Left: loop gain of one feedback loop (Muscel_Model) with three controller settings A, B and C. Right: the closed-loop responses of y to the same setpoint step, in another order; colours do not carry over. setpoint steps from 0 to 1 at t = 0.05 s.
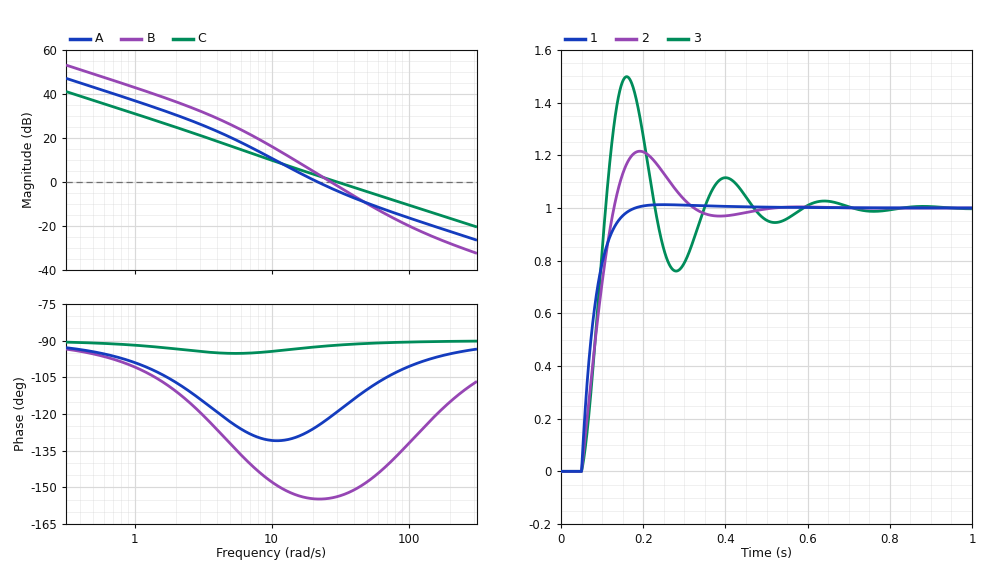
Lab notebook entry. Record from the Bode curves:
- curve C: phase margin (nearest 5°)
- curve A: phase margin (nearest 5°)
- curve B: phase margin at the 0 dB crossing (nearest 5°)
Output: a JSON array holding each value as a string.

["90°", "55°", "25°"]
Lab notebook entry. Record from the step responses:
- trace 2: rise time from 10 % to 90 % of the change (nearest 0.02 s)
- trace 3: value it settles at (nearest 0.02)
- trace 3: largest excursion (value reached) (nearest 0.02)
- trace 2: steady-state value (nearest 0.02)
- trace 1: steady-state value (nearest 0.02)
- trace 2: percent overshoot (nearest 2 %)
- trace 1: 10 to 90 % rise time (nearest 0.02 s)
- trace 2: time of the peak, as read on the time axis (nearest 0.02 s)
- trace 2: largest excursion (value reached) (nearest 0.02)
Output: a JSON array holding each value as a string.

["0.06 s", "1.00", "1.50", "1.00", "1.00", "22 %", "0.06 s", "0.20 s", "1.22"]
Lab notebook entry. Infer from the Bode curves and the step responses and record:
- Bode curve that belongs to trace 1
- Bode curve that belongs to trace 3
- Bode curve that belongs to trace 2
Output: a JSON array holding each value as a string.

["C", "B", "A"]
